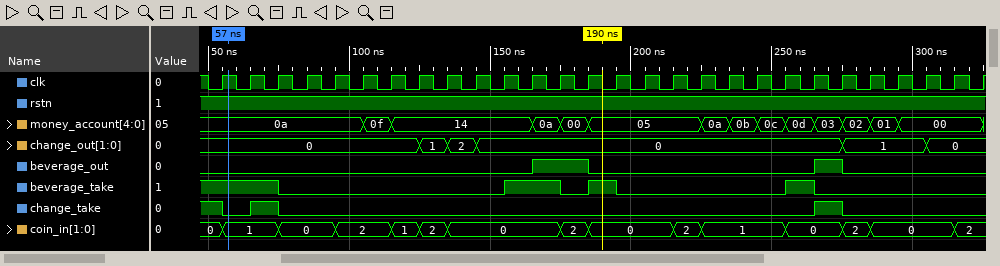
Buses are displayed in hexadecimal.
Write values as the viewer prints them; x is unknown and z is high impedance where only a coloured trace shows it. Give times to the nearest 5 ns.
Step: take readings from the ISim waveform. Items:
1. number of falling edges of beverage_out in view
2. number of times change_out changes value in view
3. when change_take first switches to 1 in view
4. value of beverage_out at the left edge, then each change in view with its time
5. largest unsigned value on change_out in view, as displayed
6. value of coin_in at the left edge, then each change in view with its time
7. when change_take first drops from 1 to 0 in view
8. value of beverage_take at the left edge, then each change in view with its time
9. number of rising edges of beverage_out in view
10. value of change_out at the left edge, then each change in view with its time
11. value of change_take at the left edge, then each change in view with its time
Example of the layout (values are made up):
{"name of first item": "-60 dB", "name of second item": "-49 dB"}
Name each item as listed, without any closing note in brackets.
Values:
{"number of falling edges of beverage_out in view": "2", "number of times change_out changes value in view": "5", "when change_take first switches to 1 in view": "65 ns", "value of beverage_out at the left edge, then each change in view with its time": "0, 1 at 165 ns, 0 at 185 ns, 1 at 265 ns, 0 at 275 ns", "largest unsigned value on change_out in view, as displayed": "2", "value of coin_in at the left edge, then each change in view with its time": "0, 1 at 55 ns, 0 at 75 ns, 2 at 95 ns, 1 at 115 ns, 2 at 125 ns, 0 at 135 ns, 2 at 175 ns, 0 at 185 ns, 2 at 215 ns, 1 at 225 ns, 0 at 255 ns, 2 at 275 ns, 0 at 285 ns, 2 at 315 ns", "when change_take first drops from 1 to 0 in view": "55 ns", "value of beverage_take at the left edge, then each change in view with its time": "1, 0 at 75 ns, 1 at 155 ns, 0 at 175 ns, 1 at 185 ns, 0 at 195 ns, 1 at 255 ns, 0 at 265 ns", "number of rising edges of beverage_out in view": "2", "value of change_out at the left edge, then each change in view with its time": "0, 1 at 125 ns, 2 at 135 ns, 0 at 145 ns, 1 at 275 ns, 0 at 305 ns", "value of change_take at the left edge, then each change in view with its time": "1, 0 at 55 ns, 1 at 65 ns, 0 at 75 ns, 1 at 265 ns, 0 at 275 ns"}
